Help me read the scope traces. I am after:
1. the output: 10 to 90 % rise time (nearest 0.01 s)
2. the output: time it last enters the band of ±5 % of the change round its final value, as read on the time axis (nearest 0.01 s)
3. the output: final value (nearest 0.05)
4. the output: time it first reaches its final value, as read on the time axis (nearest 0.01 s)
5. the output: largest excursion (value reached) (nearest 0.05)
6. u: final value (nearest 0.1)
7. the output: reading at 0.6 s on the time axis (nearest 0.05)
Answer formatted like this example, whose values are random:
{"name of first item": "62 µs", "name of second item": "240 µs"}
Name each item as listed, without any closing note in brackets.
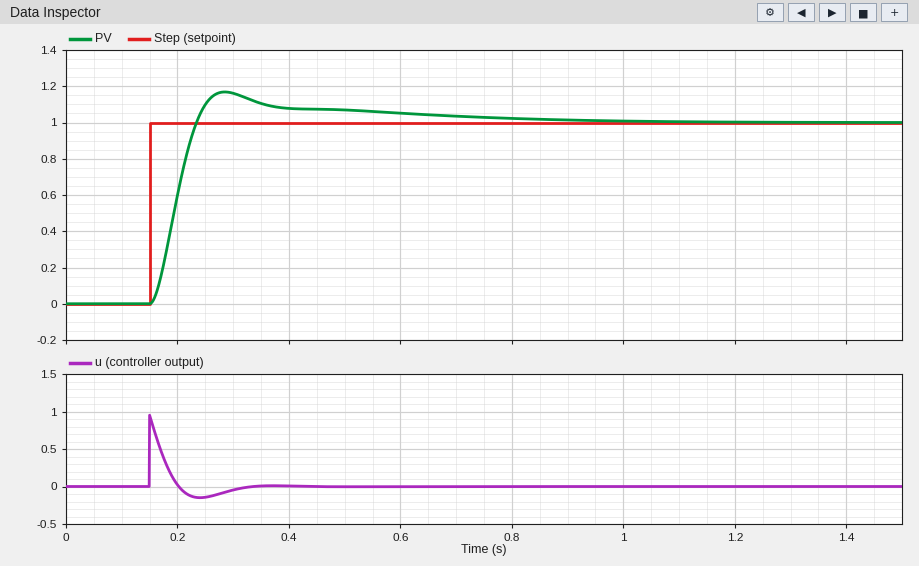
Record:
{"the output: 10 to 90 % rise time": "0.06 s", "the output: time it last enters the band of ±5 % of the change round its final value, as read on the time axis": "0.61 s", "the output: final value": "1.00", "the output: time it first reaches its final value, as read on the time axis": "0.23 s", "the output: largest excursion (value reached)": "1.15", "u: final value": "0.0", "the output: reading at 0.6 s on the time axis": "1.05"}
